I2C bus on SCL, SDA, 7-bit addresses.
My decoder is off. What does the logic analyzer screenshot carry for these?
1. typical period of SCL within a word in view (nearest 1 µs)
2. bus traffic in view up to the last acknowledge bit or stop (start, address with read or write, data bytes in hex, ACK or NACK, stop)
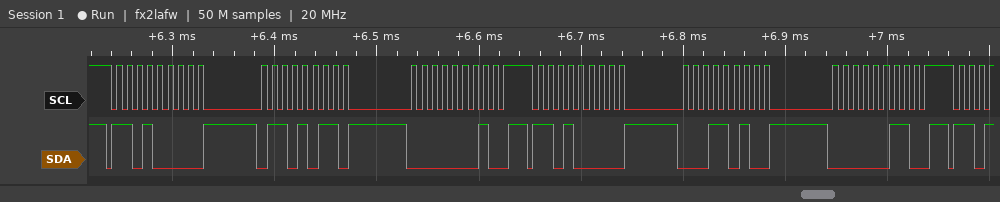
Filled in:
10 µs
start, address 68 write ACK, 6B ACK, 01 ACK, stop, start, address 68 write ACK, 1A ACK, 03 ACK, stop
